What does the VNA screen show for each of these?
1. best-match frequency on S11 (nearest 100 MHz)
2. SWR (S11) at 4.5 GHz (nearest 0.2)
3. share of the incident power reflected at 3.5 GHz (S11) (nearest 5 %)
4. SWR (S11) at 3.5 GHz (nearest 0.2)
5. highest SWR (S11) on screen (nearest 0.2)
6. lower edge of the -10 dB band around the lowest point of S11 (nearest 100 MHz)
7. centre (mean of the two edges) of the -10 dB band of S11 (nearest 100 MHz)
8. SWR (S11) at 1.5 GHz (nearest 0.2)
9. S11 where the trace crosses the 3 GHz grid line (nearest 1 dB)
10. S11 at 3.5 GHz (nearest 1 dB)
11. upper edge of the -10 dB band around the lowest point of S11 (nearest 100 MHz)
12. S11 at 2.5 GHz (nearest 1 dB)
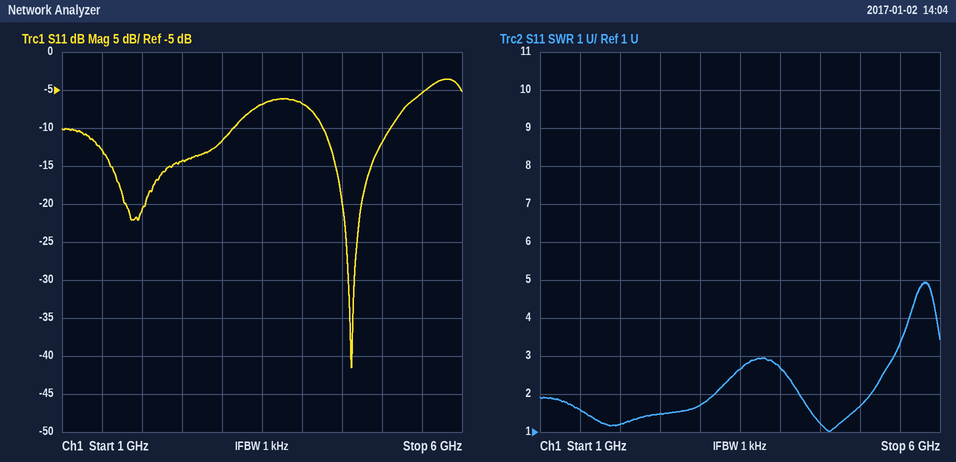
4.6 GHz
1.2
20 %
2.6
5.0
4.3 GHz
4.7 GHz
1.6
-12 dB
-7 dB
5.1 GHz
-14 dB
